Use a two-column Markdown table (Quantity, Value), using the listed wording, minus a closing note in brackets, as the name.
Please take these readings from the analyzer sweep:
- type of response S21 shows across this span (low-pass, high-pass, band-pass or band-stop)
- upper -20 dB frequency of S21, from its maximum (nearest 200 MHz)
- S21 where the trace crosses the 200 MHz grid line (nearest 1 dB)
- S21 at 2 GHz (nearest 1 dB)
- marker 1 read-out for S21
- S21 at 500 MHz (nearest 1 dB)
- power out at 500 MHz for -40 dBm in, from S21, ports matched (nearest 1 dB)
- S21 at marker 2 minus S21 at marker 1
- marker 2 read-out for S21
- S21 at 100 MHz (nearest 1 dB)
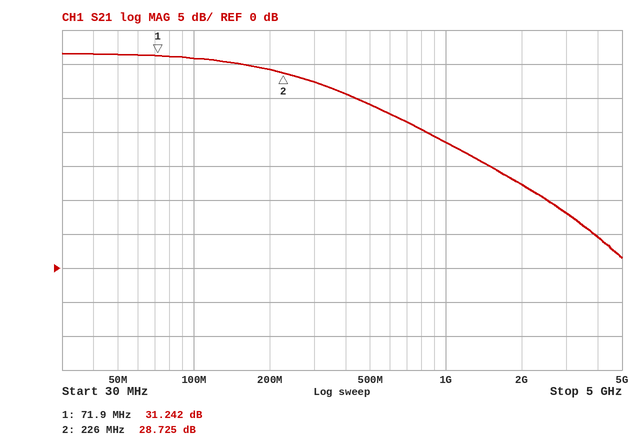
| Quantity | Value |
|---|---|
| type of response S21 shows across this span | low-pass |
| upper -20 dB frequency of S21, from its maximum | 2.2 GHz |
| S21 where the trace crosses the 200 MHz grid line | 29 dB |
| S21 at 2 GHz | 12 dB |
| marker 1 read-out for S21 | 31.242 dB |
| S21 at 500 MHz | 24 dB |
| power out at 500 MHz for -40 dBm in, from S21, ports matched | -16 dBm |
| S21 at marker 2 minus S21 at marker 1 | -2.517 dB |
| marker 2 read-out for S21 | 28.725 dB |
| S21 at 100 MHz | 31 dB |
